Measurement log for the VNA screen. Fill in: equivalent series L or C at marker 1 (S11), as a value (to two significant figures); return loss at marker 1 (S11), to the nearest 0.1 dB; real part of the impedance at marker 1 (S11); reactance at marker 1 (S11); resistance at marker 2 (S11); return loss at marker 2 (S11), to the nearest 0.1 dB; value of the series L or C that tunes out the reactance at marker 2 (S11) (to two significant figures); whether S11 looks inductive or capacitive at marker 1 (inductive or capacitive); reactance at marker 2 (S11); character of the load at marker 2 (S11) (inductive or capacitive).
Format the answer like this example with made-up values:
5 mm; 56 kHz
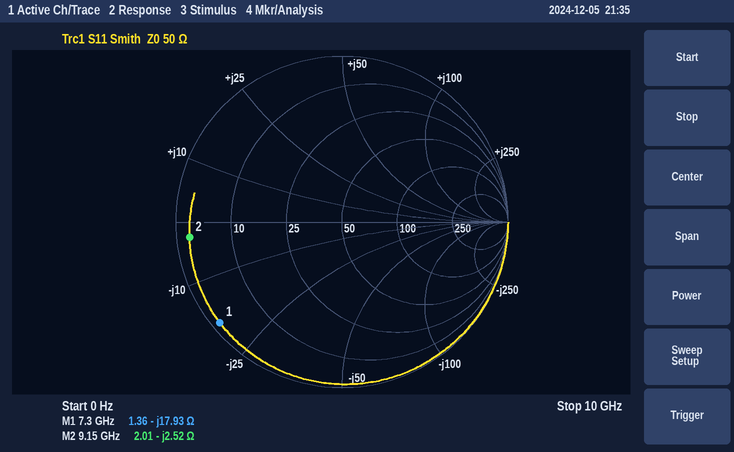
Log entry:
1.2 pF; 0.4 dB; 1.36 Ω; -17.93 Ω; 2.01 Ω; 0.7 dB; 44 pH; capacitive; -2.52 Ω; capacitive
